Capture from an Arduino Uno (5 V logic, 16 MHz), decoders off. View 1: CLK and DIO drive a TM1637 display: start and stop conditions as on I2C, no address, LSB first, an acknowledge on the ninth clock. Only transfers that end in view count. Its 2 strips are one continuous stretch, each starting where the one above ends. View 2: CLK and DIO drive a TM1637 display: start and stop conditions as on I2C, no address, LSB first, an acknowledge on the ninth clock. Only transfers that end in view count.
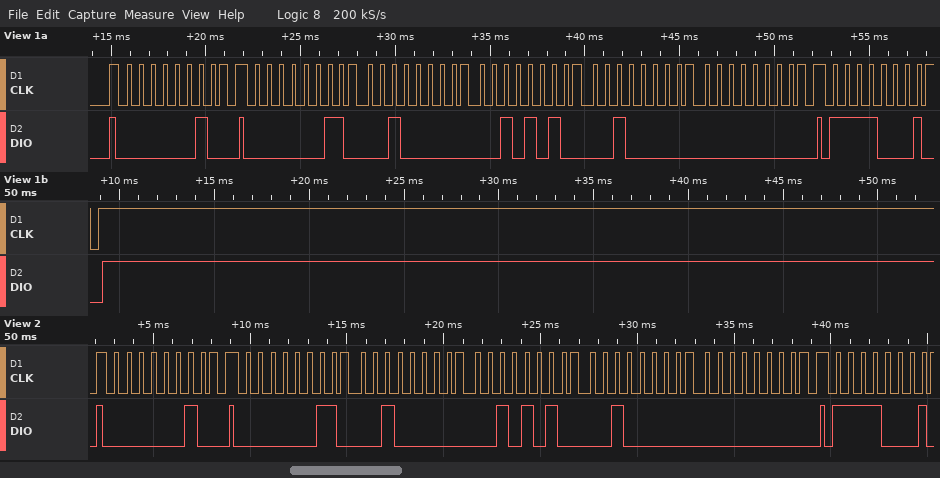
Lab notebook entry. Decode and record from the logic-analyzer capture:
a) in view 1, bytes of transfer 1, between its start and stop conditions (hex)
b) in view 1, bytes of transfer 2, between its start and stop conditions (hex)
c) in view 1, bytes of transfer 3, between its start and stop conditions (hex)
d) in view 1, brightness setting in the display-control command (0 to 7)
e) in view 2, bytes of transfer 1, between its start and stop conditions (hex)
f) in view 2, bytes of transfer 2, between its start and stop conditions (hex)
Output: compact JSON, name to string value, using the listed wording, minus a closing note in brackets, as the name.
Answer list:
{"in view 1, bytes of transfer 1, between its start and stop conditions": "40", "in view 1, bytes of transfer 2, between its start and stop conditions": "C0 04 54 04 00", "in view 1, bytes of transfer 3, between its start and stop conditions": "8F", "in view 1, brightness setting in the display-control command": "7", "in view 2, bytes of transfer 1, between its start and stop conditions": "40", "in view 2, bytes of transfer 2, between its start and stop conditions": "C0 04 54 04 00"}
